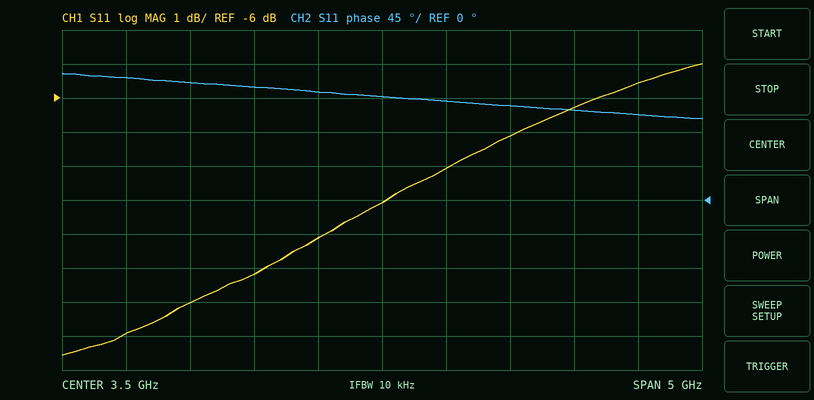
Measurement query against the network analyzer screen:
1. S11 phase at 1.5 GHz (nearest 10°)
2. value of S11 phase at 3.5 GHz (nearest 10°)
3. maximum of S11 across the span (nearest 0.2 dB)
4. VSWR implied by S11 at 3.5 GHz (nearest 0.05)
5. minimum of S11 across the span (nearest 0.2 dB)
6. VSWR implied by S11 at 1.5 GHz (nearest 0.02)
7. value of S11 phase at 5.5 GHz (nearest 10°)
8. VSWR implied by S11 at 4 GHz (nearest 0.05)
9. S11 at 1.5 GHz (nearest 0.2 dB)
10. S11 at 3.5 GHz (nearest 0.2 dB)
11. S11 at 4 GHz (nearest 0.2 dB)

160°
140°
-5.0 dB
2.10
-13.6 dB
1.58
110°
2.30
-13.0 dB
-9.0 dB
-8.0 dB
